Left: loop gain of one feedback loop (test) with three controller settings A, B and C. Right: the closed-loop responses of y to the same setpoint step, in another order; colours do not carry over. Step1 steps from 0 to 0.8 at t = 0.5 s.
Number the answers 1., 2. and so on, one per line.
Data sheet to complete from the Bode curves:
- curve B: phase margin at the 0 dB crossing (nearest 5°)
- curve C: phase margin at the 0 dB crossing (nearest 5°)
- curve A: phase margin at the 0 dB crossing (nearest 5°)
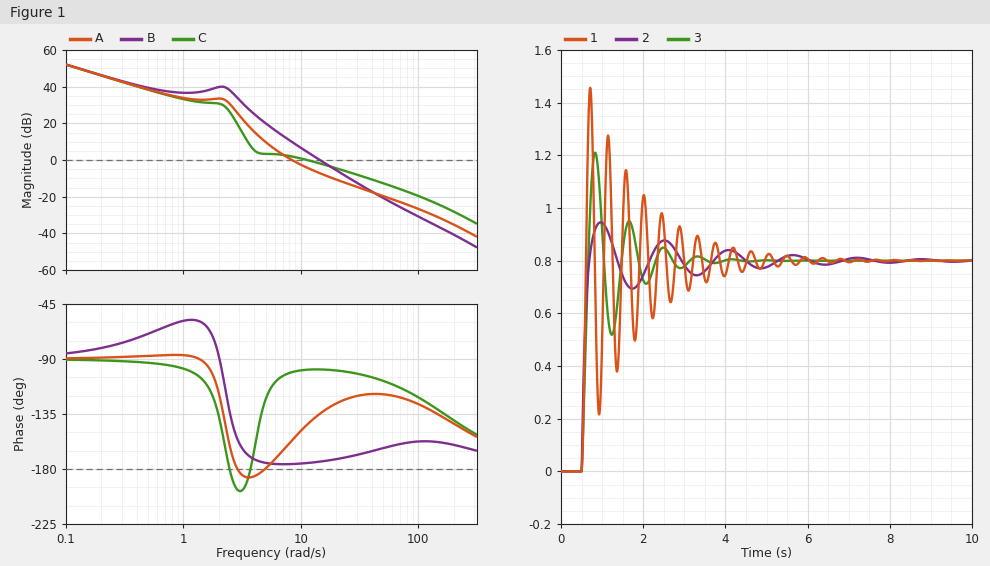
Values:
1. 5°
2. 80°
3. 25°
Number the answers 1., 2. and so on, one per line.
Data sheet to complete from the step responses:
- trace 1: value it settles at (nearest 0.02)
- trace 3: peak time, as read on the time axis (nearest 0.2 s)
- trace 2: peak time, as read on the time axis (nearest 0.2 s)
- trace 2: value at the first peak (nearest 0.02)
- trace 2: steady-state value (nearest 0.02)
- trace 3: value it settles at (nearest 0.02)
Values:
1. 0.80
2. 0.8 s
3. 1.0 s
4. 0.94
5. 0.80
6. 0.80
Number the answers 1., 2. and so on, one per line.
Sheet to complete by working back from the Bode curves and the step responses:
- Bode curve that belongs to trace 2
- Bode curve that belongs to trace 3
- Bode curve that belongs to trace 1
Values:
1. C
2. A
3. B
